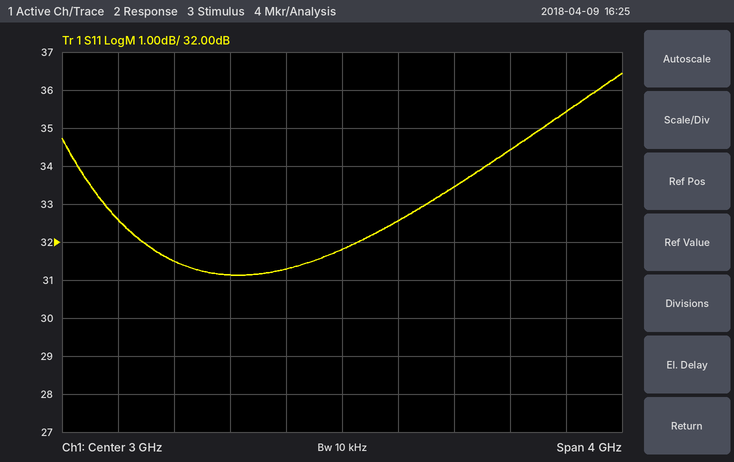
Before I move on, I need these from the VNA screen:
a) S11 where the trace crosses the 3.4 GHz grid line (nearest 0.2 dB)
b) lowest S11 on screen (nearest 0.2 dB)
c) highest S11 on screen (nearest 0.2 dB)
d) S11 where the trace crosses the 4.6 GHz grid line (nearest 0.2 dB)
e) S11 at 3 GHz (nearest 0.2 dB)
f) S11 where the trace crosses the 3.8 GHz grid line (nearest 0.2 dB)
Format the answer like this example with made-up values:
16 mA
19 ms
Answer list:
32.6 dB
31.2 dB
36.4 dB
35.4 dB
31.8 dB
33.4 dB
